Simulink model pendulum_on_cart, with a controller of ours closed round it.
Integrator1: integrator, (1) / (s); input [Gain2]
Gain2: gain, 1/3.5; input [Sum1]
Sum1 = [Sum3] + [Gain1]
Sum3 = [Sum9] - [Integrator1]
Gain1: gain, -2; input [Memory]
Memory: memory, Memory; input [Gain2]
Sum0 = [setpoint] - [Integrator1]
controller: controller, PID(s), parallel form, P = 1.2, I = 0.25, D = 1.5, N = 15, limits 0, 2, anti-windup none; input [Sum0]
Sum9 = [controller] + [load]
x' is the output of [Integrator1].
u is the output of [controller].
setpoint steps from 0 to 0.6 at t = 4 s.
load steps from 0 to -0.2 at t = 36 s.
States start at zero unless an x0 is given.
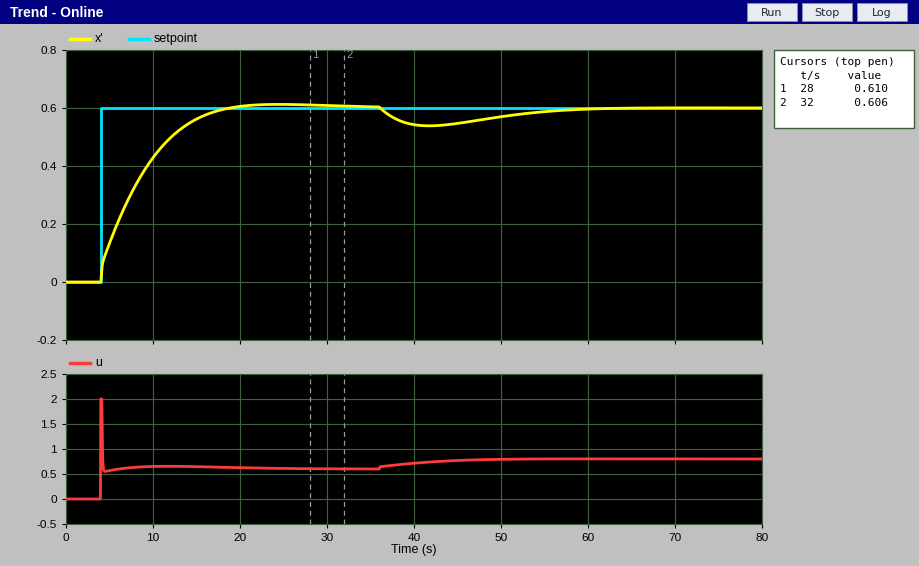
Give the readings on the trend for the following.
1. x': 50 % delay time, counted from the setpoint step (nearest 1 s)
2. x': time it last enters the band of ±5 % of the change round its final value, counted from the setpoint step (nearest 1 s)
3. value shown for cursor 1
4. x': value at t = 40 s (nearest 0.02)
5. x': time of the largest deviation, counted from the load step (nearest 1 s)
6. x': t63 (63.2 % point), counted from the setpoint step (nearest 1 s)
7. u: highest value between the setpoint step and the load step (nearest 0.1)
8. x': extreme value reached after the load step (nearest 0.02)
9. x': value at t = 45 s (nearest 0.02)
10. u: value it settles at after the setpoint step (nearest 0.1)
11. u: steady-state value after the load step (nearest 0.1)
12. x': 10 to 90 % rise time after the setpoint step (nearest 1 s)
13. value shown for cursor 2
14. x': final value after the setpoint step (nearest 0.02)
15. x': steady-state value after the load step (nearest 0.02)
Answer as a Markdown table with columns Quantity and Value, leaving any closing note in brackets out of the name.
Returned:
| Quantity | Value |
|---|---|
| x': 50 % delay time, counted from the setpoint step | 3 s |
| x': time it last enters the band of ±5 % of the change round its final value, counted from the setpoint step | 12 s |
| value shown for cursor 1 | 0.610 |
| x': value at t = 40 s | 0.54 |
| x': time of the largest deviation, counted from the load step | 6 s |
| x': t63 (63.2 % point), counted from the setpoint step | 5 s |
| u: highest value between the setpoint step and the load step | 2.0 |
| x': extreme value reached after the load step | 0.54 |
| x': value at t = 45 s | 0.54 |
| u: value it settles at after the setpoint step | 0.6 |
| u: steady-state value after the load step | 0.8 |
| x': 10 to 90 % rise time after the setpoint step | 10 s |
| value shown for cursor 2 | 0.606 |
| x': final value after the setpoint step | 0.60 |
| x': steady-state value after the load step | 0.60 |
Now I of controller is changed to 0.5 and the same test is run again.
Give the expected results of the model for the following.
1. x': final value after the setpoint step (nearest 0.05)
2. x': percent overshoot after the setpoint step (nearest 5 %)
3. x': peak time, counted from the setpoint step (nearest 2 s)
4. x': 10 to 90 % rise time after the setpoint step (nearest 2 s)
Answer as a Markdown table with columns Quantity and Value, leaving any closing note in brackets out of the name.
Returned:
| Quantity | Value |
|---|---|
| x': final value after the setpoint step | 0.60 |
| x': percent overshoot after the setpoint step | 10 % |
| x': peak time, counted from the setpoint step | 12 s |
| x': 10 to 90 % rise time after the setpoint step | 6 s |
